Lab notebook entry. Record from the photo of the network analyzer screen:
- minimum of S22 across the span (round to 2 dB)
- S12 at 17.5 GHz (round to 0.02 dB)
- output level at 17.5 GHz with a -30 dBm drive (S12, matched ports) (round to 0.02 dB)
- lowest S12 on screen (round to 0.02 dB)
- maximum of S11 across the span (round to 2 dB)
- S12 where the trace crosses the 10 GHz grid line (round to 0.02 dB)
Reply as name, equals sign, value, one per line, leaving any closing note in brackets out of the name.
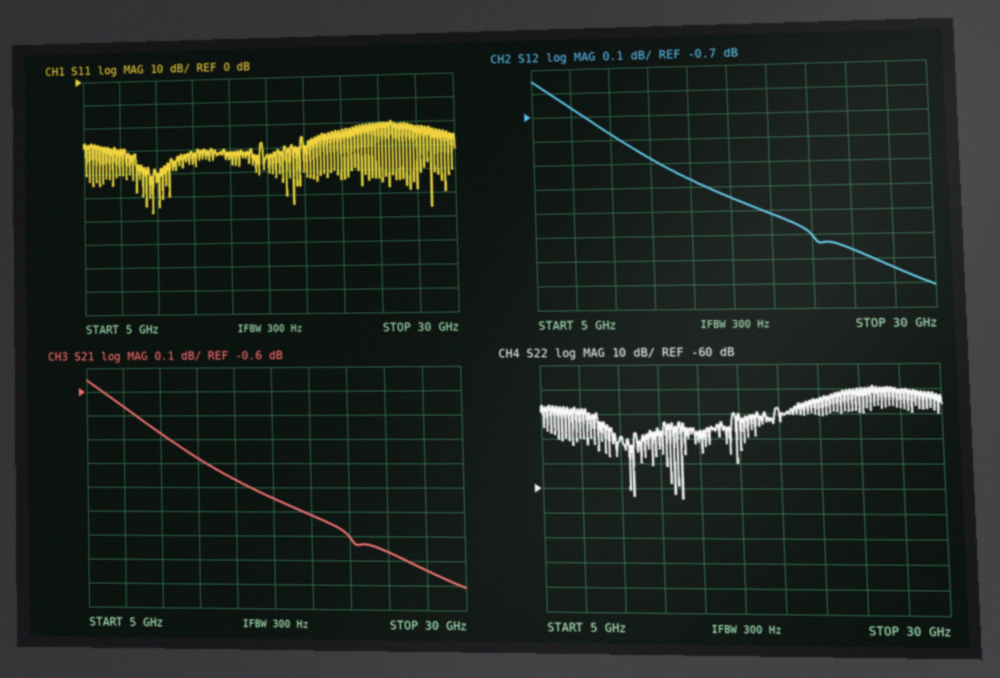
minimum of S22 across the span = -64 dB
S12 at 17.5 GHz = -1.04 dB
output level at 17.5 GHz with a -30 dBm drive (S12, matched ports) = -31.04 dBm
lowest S12 on screen = -1.40 dB
maximum of S11 across the span = -20 dB
S12 where the trace crosses the 10 GHz grid line = -0.78 dB
